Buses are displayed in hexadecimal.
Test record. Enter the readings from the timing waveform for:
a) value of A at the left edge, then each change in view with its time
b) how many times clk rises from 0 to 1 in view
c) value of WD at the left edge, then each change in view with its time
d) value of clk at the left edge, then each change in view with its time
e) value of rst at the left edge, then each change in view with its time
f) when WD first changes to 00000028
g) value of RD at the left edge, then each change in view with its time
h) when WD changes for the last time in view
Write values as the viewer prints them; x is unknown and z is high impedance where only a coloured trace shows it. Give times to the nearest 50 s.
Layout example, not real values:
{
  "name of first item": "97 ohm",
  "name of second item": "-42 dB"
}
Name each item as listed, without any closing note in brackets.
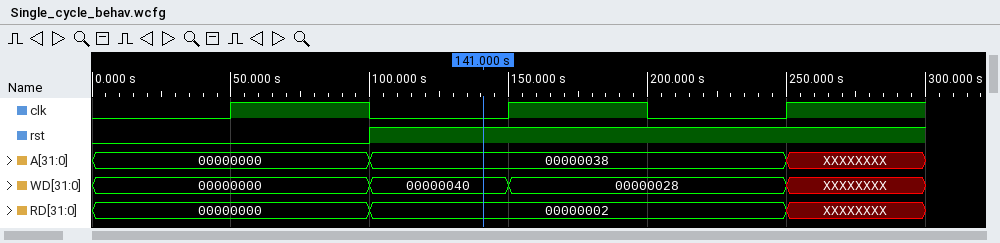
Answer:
{
  "value of A at the left edge, then each change in view with its time": "00000000, 00000038 at 100 s, XXXXXXXX at 250 s",
  "how many times clk rises from 0 to 1 in view": "3",
  "value of WD at the left edge, then each change in view with its time": "00000000, 00000040 at 100 s, 00000028 at 150 s, XXXXXXXX at 250 s",
  "value of clk at the left edge, then each change in view with its time": "0, 1 at 50 s, 0 at 100 s, 1 at 150 s, 0 at 200 s, 1 at 250 s",
  "value of rst at the left edge, then each change in view with its time": "0, 1 at 100 s",
  "when WD first changes to 00000028": "150 s",
  "value of RD at the left edge, then each change in view with its time": "00000000, 00000002 at 100 s, XXXXXXXX at 250 s",
  "when WD changes for the last time in view": "250 s"
}
